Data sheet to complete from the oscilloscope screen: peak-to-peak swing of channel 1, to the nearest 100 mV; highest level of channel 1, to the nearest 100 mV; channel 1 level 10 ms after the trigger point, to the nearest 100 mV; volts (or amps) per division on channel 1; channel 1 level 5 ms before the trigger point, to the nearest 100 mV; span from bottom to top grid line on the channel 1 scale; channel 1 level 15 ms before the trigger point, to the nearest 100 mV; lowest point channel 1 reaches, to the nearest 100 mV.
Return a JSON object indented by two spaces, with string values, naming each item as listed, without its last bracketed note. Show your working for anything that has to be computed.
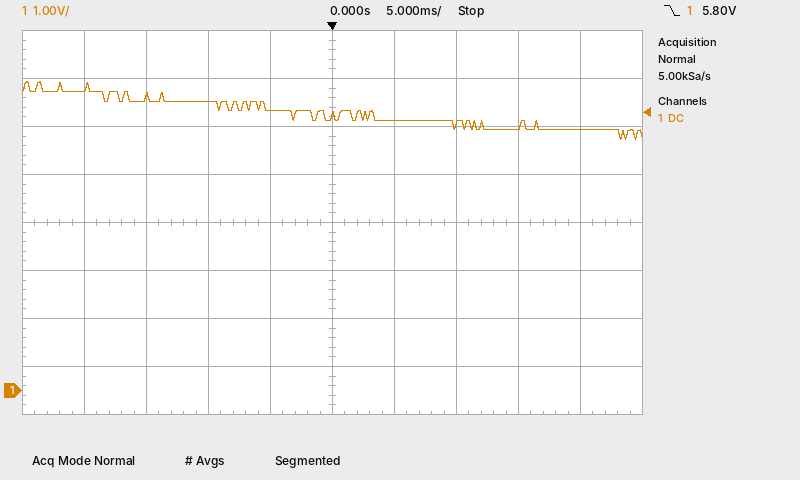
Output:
{
  "peak-to-peak swing of channel 1, to the nearest 100 mV": "6.4 V − (5.2 V) = 1.2 V",
  "highest level of channel 1, to the nearest 100 mV": "6.4 V",
  "channel 1 level 10 ms after the trigger point, to the nearest 100 mV": "5.5 V",
  "volts (or amps) per division on channel 1": "1 V",
  "channel 1 level 5 ms before the trigger point, to the nearest 100 mV": "5.8 V",
  "span from bottom to top grid line on the channel 1 scale": "8 V",
  "channel 1 level 15 ms before the trigger point, to the nearest 100 mV": "6.1 V",
  "lowest point channel 1 reaches, to the nearest 100 mV": "5.2 V"
}
